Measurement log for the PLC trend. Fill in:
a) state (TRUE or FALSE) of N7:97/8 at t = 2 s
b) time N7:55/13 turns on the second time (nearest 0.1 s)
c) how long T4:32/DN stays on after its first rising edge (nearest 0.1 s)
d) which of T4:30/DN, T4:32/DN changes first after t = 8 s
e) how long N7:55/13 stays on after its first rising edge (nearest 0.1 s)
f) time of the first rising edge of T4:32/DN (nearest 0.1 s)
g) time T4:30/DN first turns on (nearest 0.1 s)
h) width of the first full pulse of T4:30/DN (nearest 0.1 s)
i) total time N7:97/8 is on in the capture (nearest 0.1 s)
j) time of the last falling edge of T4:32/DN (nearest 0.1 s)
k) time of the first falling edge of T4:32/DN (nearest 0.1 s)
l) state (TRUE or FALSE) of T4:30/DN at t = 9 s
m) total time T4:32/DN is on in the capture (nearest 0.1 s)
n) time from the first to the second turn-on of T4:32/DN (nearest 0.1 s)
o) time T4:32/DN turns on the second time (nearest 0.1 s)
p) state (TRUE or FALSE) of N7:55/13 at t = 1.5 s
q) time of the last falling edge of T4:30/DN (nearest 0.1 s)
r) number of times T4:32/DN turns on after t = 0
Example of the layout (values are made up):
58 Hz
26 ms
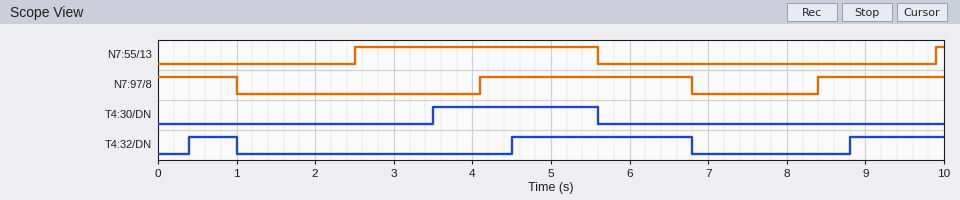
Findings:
FALSE
9.9 s
0.6 s
T4:32/DN
3.1 s
0.4 s
3.5 s
2.1 s
5.3 s
6.8 s
1.0 s
FALSE
4.1 s
4.1 s
4.5 s
FALSE
5.6 s
3
